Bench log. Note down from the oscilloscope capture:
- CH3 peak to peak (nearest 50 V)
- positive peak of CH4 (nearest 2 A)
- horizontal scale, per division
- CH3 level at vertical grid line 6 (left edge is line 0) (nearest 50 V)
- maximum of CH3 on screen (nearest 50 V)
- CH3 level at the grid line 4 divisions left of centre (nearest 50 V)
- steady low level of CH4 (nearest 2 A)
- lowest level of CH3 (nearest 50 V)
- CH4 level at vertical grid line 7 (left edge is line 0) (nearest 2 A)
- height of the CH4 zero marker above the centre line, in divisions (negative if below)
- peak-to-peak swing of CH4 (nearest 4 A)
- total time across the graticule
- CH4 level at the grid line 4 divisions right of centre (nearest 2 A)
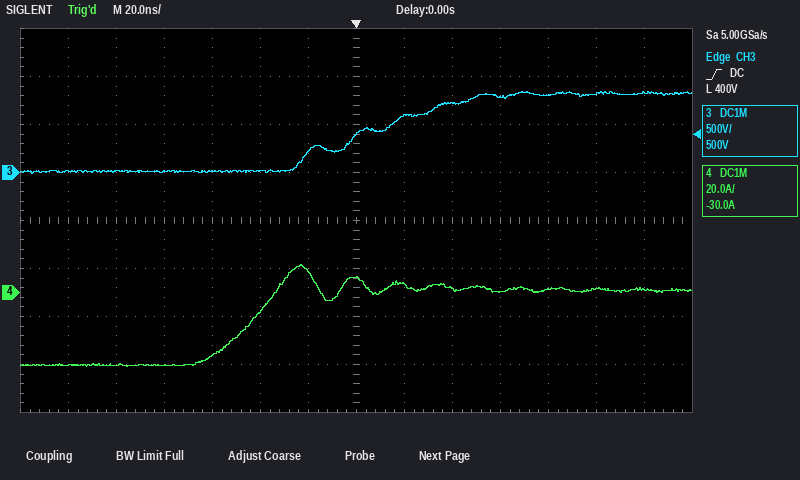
850 V
12 A
20 ns
200 V
850 V
0 V
-30 A
0 V
6 A
-1.5 div
44 A
280 ns
2 A
